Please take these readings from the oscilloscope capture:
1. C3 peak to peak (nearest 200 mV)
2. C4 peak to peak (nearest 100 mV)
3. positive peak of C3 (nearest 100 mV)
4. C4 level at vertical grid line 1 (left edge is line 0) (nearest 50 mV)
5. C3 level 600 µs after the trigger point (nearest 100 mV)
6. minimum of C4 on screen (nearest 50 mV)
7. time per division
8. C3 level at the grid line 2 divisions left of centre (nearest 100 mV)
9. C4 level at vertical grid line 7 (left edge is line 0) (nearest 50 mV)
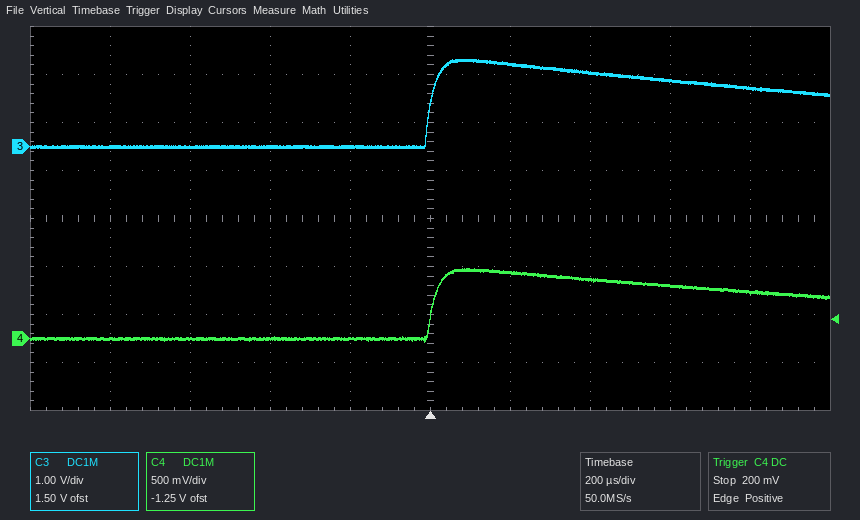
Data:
1.8 V
800 mV
1.8 V
0 mV
1.4 V
-50 mV
200 µs
0.0 V
600 mV
